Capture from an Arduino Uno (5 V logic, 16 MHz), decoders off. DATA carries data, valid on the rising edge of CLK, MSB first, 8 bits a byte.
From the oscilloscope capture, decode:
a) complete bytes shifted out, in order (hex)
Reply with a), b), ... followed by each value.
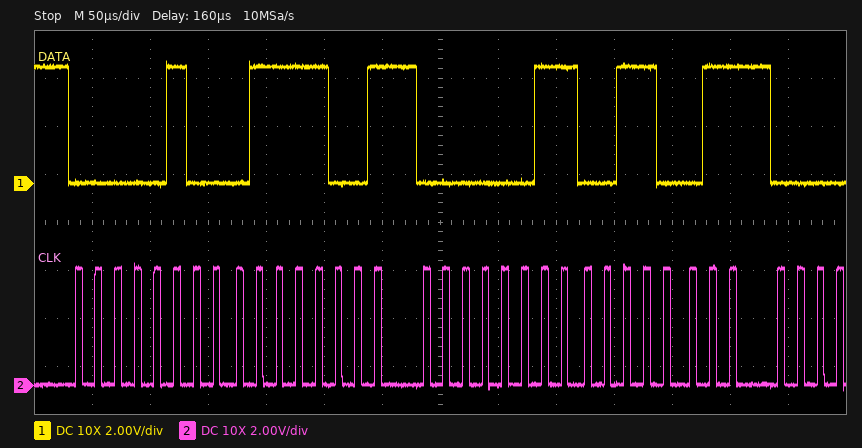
a) 0x04 0x79 0x03 0x33
